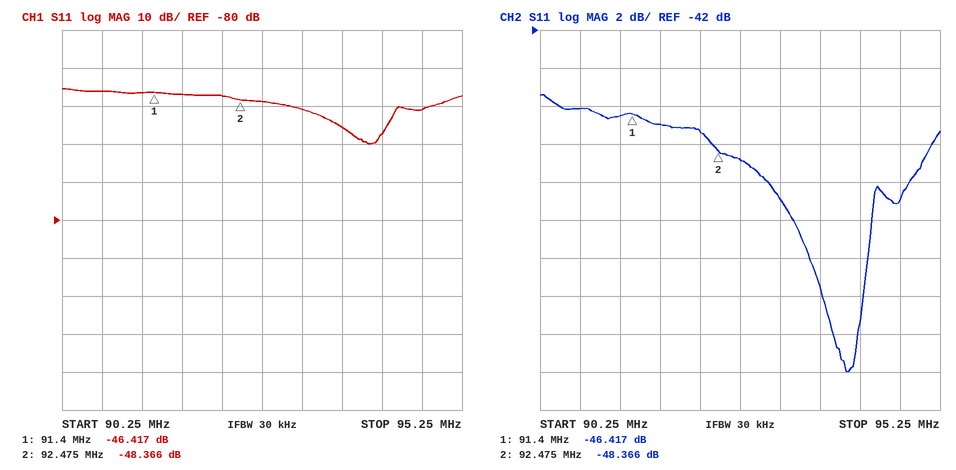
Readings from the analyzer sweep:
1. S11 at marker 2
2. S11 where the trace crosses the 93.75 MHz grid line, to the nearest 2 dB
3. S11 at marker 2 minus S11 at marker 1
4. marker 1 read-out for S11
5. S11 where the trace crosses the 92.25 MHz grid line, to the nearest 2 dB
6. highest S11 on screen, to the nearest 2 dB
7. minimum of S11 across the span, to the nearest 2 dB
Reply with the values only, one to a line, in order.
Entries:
-48.366 dB
-56 dB
-1.949 dB
-46.417 dB
-48 dB
-46 dB
-60 dB
